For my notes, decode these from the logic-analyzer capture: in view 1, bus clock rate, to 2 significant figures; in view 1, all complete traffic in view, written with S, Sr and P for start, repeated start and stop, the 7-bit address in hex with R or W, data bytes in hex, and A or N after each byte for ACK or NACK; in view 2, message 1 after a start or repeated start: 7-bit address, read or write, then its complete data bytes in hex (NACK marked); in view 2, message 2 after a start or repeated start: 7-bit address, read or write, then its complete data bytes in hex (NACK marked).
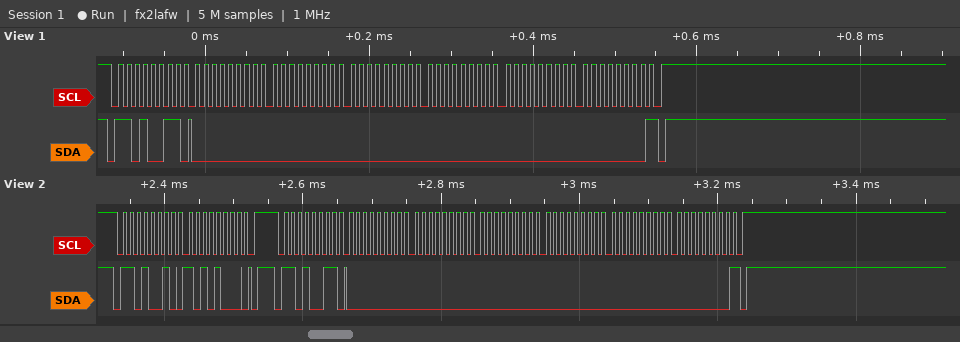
100 kHz
S 69R A 00 A 00 A 00 A 00 A 00 A 00 N P
0x69 write: A8
0x69 read: 00 00 00 00 00 00 NACK
